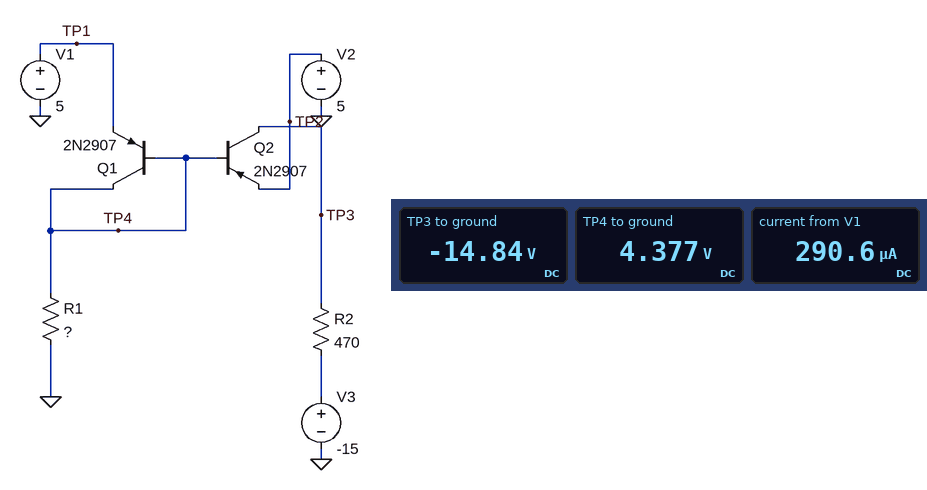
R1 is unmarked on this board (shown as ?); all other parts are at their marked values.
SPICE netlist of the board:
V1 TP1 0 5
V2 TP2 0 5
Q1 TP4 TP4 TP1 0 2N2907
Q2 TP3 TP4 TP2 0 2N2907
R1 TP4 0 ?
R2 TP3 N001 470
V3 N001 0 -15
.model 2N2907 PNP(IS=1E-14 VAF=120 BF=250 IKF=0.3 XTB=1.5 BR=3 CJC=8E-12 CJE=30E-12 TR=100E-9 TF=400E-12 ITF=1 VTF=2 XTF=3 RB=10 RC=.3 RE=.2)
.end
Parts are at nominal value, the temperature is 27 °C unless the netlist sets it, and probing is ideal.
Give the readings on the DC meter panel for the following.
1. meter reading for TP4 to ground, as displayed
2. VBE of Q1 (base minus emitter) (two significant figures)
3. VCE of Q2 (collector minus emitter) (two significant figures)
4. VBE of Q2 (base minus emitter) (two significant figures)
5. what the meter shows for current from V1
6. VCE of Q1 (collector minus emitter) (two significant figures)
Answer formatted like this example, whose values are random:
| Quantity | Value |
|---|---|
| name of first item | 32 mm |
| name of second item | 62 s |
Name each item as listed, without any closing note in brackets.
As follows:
| Quantity | Value |
|---|---|
| meter reading for TP4 to ground, as displayed | 4.377 V |
| VBE of Q1 (base minus emitter) | -620 mV |
| VCE of Q2 (collector minus emitter) | -20 V |
| VBE of Q2 (base minus emitter) | -620 mV |
| what the meter shows for current from V1 | 290.6 µA |
| VCE of Q1 (collector minus emitter) | -620 mV |
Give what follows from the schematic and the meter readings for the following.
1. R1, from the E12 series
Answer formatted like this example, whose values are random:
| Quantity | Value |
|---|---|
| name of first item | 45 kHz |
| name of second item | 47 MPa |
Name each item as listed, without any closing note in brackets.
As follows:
| Quantity | Value |
|---|---|
| R1, from the E12 series | 15 kΩ |
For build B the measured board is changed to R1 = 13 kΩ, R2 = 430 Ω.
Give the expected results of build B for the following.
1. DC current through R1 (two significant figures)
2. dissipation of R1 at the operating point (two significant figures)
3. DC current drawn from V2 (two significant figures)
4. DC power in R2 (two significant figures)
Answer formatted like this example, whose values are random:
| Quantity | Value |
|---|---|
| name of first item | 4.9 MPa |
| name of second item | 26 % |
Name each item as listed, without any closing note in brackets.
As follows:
| Quantity | Value |
|---|---|
| DC current through R1 | 340 µA |
| dissipation of R1 at the operating point | 1.5 mW |
| DC current drawn from V2 | 390 µA |
| DC power in R2 | 64 µW |
